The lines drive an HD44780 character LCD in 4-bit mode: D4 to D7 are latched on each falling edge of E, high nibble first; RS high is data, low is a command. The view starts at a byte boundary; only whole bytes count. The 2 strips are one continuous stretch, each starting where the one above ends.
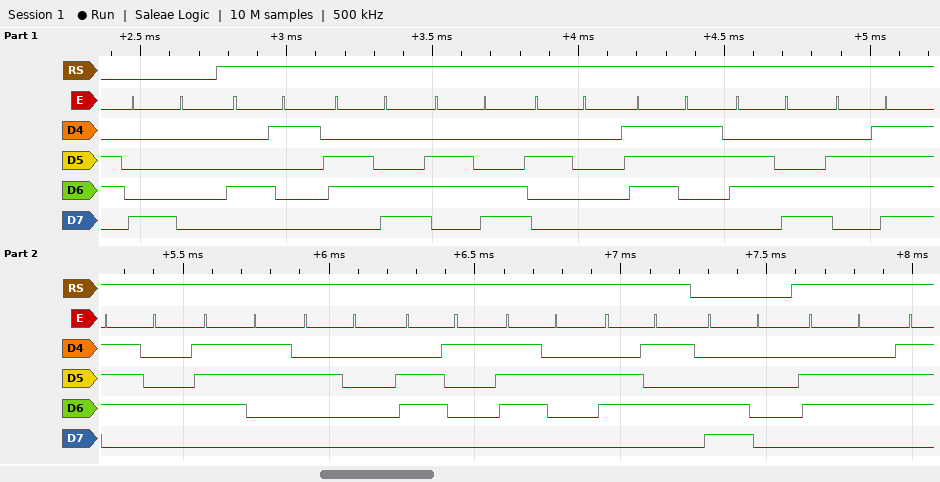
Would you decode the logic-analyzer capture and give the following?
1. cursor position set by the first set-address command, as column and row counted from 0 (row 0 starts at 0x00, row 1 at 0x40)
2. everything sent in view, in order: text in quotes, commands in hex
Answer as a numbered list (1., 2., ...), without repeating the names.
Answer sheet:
1. column 0, row 0
2. 0x80 "All slots are" 0xC0 "f"
